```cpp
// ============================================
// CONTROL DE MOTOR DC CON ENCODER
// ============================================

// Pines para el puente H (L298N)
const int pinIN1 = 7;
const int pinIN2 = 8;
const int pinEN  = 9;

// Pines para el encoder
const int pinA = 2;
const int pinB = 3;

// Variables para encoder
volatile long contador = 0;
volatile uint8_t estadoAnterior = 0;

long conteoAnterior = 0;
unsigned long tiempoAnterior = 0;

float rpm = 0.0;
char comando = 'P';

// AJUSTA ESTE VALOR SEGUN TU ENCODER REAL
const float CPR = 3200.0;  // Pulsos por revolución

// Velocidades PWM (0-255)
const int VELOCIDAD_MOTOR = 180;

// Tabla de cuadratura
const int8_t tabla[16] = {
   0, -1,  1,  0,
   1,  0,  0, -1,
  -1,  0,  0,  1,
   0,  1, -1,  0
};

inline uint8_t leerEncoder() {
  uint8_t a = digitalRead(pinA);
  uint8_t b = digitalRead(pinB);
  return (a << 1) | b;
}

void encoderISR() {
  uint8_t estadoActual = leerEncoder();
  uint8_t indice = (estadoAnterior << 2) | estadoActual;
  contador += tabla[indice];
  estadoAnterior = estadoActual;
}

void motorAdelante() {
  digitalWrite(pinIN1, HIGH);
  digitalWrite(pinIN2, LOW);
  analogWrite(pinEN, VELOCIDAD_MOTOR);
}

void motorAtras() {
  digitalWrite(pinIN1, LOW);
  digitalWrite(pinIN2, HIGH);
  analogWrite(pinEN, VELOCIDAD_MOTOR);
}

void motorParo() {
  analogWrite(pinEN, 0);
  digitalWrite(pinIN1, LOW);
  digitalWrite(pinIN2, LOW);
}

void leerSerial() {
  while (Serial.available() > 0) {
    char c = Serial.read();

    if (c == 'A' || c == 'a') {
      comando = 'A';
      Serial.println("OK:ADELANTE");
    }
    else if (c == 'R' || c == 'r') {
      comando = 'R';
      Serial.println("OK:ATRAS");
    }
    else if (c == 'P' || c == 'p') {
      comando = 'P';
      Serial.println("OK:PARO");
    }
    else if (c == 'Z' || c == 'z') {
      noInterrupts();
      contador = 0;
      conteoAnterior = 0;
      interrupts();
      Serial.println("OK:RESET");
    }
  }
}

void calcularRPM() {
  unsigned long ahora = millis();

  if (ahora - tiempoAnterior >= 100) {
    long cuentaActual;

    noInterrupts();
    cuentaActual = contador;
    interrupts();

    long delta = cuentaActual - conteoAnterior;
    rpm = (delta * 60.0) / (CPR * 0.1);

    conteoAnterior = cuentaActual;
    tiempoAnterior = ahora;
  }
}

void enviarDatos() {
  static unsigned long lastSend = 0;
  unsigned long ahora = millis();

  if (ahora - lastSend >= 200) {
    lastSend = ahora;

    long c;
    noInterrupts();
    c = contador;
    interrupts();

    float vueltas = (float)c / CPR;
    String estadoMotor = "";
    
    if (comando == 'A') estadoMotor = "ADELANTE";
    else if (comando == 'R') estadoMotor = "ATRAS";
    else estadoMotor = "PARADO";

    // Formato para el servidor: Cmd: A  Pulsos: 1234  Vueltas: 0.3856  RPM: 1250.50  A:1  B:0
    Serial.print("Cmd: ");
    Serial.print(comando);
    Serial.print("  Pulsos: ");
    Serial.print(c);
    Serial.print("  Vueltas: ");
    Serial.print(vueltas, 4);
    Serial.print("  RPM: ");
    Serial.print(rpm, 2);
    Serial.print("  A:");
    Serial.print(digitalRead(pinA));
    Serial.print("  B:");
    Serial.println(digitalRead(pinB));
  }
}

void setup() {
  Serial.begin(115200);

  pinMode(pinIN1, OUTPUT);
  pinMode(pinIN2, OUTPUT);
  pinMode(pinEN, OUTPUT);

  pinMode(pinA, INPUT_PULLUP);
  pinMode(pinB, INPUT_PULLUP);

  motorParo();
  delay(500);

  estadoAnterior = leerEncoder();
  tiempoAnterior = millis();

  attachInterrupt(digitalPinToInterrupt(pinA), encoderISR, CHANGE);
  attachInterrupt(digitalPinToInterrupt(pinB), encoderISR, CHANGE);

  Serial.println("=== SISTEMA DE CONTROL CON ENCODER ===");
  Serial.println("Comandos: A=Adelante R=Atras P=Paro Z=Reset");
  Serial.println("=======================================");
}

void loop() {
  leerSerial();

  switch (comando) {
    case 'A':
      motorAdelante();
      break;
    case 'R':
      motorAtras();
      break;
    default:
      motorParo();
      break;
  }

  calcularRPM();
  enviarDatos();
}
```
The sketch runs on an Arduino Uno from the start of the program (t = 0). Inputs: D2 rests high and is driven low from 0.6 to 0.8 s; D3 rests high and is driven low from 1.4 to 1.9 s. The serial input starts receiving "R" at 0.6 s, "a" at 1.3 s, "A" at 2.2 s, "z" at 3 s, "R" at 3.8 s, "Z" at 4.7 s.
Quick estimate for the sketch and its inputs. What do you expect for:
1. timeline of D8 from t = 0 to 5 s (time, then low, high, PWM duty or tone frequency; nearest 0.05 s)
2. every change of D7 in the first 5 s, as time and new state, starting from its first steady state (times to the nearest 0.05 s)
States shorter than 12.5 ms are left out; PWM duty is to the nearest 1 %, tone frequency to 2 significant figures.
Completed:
0 s low; 0.6 s high; 1.3 s low; 3.8 s high
0 s low; 1.3 s high; 3.8 s low
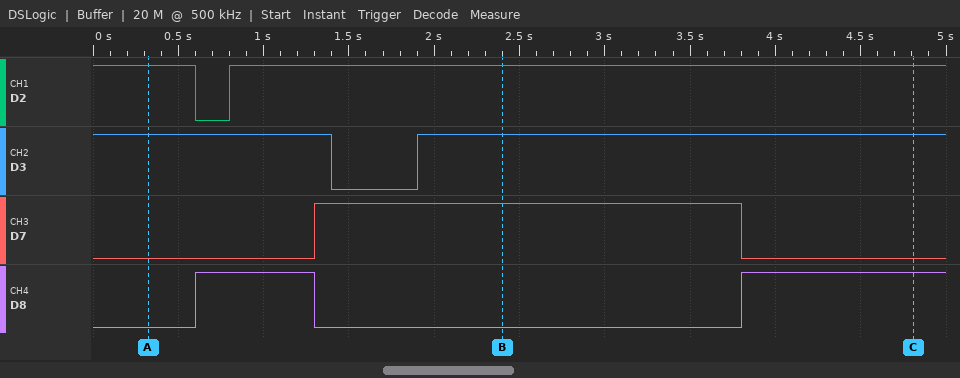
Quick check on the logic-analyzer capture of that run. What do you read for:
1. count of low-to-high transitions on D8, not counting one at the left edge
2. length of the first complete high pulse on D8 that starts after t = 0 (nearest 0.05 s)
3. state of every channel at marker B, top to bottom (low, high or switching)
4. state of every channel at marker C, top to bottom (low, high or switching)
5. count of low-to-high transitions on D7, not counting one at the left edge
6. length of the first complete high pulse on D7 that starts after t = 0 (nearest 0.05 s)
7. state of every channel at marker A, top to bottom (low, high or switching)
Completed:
2
0.70 s
D2 high, D3 high, D7 high, D8 low
D2 high, D3 high, D7 low, D8 high
1
2.50 s
D2 high, D3 high, D7 low, D8 low
